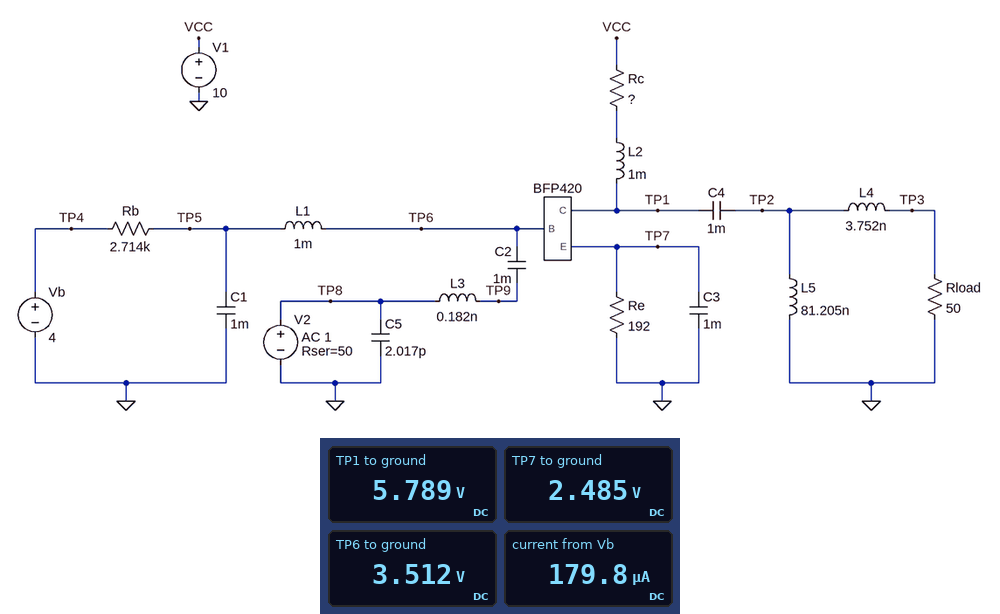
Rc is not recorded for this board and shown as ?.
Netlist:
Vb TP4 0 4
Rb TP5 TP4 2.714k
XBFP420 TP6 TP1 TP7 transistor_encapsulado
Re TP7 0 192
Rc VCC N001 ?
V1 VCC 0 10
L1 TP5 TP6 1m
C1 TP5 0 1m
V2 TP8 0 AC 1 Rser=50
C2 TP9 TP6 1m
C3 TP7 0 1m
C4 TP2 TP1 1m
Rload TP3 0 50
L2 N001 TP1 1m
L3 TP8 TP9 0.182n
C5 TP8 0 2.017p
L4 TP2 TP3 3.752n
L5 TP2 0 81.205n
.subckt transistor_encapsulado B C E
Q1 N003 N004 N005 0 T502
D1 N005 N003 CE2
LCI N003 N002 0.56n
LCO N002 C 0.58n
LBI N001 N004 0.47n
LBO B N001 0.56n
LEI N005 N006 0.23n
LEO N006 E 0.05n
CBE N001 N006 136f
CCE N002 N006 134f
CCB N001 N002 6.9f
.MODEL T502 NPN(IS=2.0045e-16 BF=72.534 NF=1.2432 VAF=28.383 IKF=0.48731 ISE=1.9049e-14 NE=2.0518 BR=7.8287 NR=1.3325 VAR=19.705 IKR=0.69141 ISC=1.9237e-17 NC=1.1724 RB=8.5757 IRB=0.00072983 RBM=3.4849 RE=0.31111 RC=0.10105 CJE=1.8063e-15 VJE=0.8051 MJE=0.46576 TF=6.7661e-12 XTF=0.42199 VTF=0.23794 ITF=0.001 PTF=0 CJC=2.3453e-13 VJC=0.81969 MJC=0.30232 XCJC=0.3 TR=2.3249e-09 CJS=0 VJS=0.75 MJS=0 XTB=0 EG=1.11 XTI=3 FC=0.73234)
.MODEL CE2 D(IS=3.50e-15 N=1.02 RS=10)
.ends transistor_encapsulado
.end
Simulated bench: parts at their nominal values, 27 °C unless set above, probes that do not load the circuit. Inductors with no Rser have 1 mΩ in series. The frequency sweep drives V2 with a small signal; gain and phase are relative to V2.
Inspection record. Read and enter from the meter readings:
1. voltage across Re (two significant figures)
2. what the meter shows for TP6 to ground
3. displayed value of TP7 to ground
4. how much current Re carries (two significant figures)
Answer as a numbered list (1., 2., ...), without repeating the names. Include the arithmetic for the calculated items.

1. 2.485 V = 2.5 V
2. 3.512 V
3. 2.485 V
4. (2.485 V) / 192 Ω = 13 mA
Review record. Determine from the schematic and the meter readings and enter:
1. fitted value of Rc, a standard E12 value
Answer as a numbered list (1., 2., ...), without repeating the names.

1. 330 Ω
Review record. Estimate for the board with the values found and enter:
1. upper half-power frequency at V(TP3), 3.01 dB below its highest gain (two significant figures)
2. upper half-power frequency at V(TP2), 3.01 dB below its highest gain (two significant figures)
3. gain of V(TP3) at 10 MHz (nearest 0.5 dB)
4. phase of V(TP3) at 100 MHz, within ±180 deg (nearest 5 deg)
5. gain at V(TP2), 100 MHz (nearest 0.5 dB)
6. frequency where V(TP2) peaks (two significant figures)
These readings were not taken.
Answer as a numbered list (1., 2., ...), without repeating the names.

1. 650 MHz
2. 700 MHz
3. 2.5 dB
4. -150 deg
5. 19.5 dB
6. 220 MHz
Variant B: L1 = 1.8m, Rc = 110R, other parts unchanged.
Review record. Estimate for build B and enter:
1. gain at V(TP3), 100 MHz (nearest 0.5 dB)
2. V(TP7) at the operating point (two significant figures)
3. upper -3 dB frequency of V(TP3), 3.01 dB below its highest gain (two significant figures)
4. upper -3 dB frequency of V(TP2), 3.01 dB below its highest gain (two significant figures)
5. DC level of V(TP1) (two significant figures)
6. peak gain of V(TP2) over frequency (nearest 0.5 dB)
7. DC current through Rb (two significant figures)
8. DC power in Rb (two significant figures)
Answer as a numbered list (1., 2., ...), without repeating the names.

1. 20.0 dB
2. 2.5 V
3. 670 MHz
4. 720 MHz
5. 8.6 V
6. 21.5 dB
7. 170 µA
8. 76 µW
